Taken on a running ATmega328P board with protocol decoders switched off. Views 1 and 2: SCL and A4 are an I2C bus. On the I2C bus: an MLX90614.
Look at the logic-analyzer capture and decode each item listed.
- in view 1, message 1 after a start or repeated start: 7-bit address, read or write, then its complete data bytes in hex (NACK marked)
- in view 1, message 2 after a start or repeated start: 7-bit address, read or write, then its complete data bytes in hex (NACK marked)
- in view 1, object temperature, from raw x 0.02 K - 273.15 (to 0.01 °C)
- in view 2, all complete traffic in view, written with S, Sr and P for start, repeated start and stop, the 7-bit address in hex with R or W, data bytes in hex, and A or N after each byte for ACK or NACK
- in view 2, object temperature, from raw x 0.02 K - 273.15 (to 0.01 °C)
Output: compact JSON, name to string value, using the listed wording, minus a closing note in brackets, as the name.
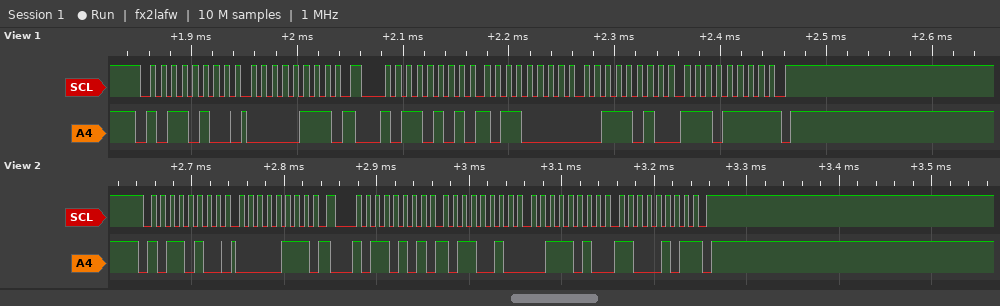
{"in view 1, message 1 after a start or repeated start: 7-bit address, read or write, then its complete data bytes in hex": "0x5A write: 07", "in view 1, message 2 after a start or repeated start: 7-bit address, read or write, then its complete data bytes in hex": "0x5A read: B0 3A EF NACK", "in view 1, object temperature, from raw x 0.02 K - 273.15": "27.33 °C", "in view 2, all complete traffic in view, written with S, Sr and P for start, repeated start and stop, the 7-bit address in hex with R or W, data bytes in hex, and A or N after each byte for ACK or NACK": "S 5AW A 07 A Sr 5AR A B2 A 3A A C5 N P", "in view 2, object temperature, from raw x 0.02 K - 273.15": "27.37 °C"}
